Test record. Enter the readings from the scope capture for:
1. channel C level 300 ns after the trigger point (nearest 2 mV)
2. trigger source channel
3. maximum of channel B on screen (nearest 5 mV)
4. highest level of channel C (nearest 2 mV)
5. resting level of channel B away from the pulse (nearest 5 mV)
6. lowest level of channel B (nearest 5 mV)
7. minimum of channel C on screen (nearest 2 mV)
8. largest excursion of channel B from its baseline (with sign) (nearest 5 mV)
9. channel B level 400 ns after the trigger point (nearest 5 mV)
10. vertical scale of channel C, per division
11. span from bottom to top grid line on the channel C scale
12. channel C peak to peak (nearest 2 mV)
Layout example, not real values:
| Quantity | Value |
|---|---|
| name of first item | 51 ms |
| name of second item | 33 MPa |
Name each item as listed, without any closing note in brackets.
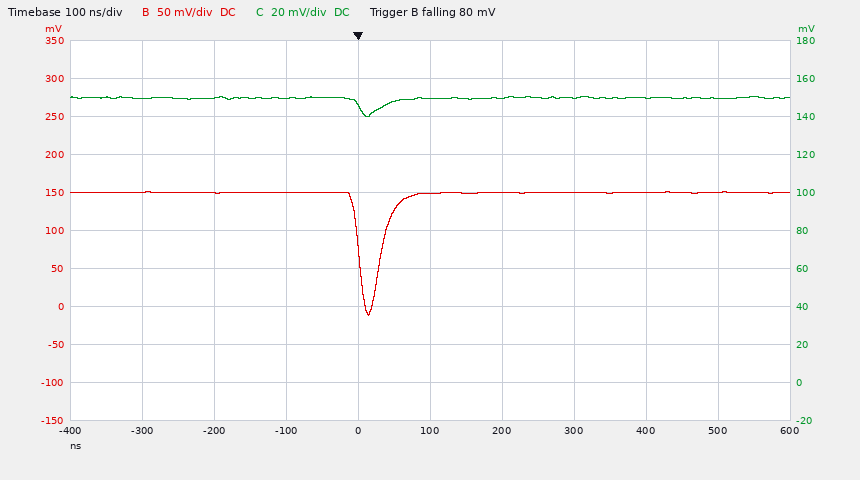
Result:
| Quantity | Value |
|---|---|
| channel C level 300 ns after the trigger point | 150 mV |
| trigger source channel | channel B |
| maximum of channel B on screen | 150 mV |
| highest level of channel C | 150 mV |
| resting level of channel B away from the pulse | 150 mV |
| lowest level of channel B | -10 mV |
| minimum of channel C on screen | 140 mV |
| largest excursion of channel B from its baseline (with sign) | -160 mV |
| channel B level 400 ns after the trigger point | 150 mV |
| vertical scale of channel C, per division | 20 mV |
| span from bottom to top grid line on the channel C scale | 200 mV |
| channel C peak to peak | 10 mV |
